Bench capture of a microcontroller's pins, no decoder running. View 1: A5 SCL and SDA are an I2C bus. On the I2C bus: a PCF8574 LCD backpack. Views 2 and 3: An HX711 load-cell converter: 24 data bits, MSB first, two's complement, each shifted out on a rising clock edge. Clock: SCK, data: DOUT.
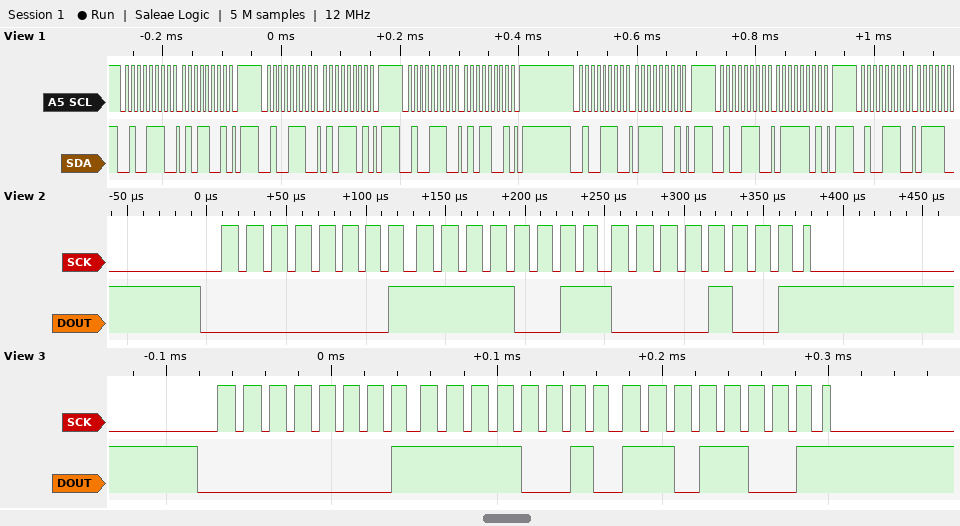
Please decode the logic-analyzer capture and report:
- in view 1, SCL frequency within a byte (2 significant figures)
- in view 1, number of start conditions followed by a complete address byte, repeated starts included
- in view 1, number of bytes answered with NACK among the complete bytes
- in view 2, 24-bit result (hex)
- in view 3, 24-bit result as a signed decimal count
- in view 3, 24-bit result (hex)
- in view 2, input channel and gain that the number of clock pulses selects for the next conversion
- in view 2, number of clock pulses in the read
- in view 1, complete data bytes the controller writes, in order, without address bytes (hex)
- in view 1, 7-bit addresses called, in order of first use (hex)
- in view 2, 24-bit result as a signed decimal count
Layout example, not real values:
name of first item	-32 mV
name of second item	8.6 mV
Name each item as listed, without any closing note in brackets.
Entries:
in view 1, SCL frequency within a byte	100 kHz
in view 1, number of start conditions followed by a complete address byte, repeated starts included	6
in view 1, number of bytes answered with NACK among the complete bytes	0
in view 2, 24-bit result	0x01F309
in view 3, 24-bit result as a signed decimal count	127705
in view 3, 24-bit result	0x01F2D9
in view 2, input channel and gain that the number of clock pulses selects for the next conversion	channel A, gain 128
in view 2, number of clock pulses in the read	25
in view 1, complete data bytes the controller writes, in order, without address bytes	59 5D 59 79 7D
in view 1, 7-bit addresses called, in order of first use	0x27
in view 2, 24-bit result as a signed decimal count	127753
